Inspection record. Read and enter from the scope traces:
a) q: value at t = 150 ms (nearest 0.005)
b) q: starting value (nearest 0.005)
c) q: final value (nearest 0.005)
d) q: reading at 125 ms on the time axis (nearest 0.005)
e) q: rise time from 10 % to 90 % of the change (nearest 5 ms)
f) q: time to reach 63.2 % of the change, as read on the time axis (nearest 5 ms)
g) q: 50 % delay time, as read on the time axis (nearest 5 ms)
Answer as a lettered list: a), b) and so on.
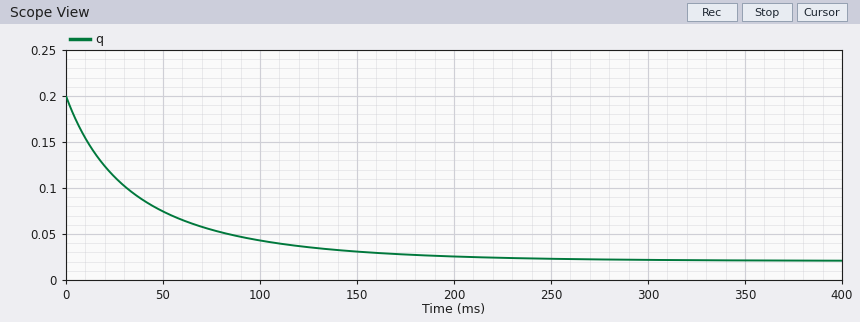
a) 0.030
b) 0.200
c) 0.020
d) 0.035
e) 110 ms
f) 40 ms
g) 25 ms
